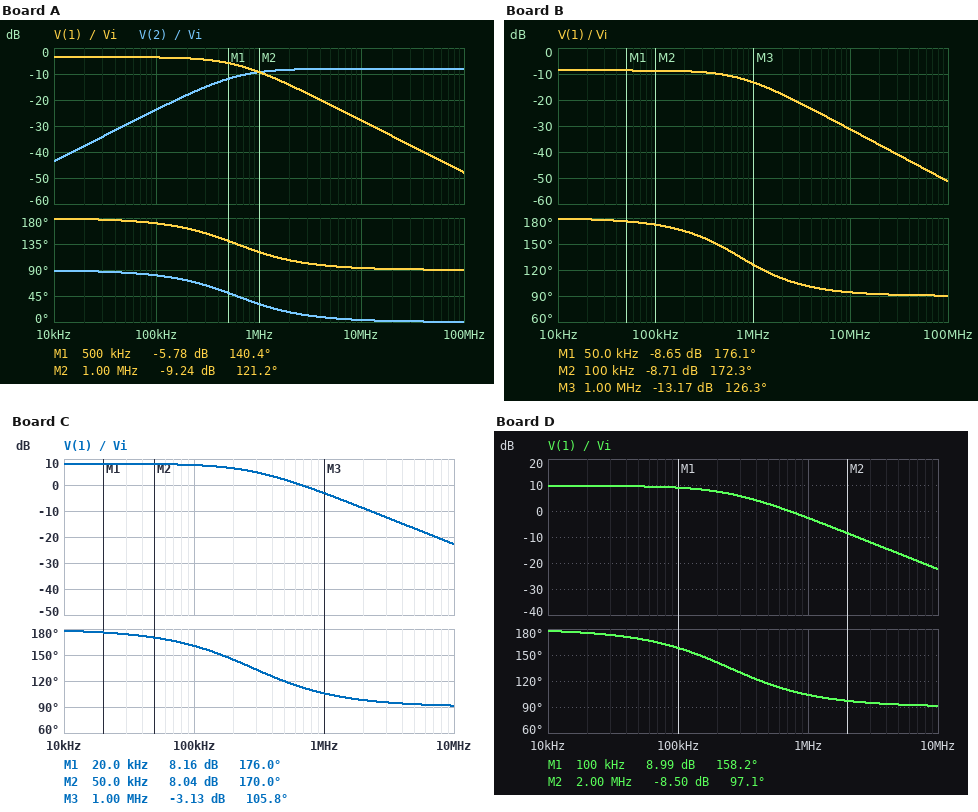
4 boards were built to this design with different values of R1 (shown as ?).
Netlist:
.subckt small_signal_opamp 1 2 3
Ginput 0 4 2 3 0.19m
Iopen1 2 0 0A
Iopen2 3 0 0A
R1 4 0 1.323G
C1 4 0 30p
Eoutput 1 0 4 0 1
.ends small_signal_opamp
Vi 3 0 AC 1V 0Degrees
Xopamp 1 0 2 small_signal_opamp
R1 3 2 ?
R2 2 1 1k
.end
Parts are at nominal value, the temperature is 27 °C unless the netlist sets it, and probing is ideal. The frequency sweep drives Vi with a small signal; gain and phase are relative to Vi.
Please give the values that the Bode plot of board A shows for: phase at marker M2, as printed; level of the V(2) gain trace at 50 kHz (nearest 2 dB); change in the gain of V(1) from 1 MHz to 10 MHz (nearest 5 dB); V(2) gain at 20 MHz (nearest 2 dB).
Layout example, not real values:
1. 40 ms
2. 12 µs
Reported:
1. 121.2 deg
2. -30 dB
3. -20 dB
4. -8 dB
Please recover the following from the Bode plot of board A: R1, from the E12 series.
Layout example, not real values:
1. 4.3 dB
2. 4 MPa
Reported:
1. 1.5 kΩ
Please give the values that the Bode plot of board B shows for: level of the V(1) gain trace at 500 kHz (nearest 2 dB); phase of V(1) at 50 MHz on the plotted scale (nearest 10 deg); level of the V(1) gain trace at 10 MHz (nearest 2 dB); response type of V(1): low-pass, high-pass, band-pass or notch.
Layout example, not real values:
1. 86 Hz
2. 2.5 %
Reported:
1. -10 dB
2. 90 deg
3. -32 dB
4. low-pass
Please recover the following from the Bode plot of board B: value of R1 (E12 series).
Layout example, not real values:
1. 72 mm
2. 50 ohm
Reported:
1. 2.7 kΩ
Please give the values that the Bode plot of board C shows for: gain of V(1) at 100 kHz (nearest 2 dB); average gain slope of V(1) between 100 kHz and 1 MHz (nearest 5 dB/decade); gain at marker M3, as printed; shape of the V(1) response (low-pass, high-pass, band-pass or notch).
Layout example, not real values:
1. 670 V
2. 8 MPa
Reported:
1. 8 dB
2. -10 dB/decade
3. -3.13 dB
4. low-pass
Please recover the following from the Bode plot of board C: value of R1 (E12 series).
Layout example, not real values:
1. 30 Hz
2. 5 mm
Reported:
1. 390 Ω
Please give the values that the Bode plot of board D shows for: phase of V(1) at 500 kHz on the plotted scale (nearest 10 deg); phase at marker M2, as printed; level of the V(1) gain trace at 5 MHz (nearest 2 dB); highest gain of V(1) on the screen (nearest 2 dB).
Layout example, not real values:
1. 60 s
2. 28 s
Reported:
1. 120 deg
2. 97.1 deg
3. -16 dB
4. 10 dB
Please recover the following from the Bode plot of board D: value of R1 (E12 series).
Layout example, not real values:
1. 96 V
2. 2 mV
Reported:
1. 330 Ω
